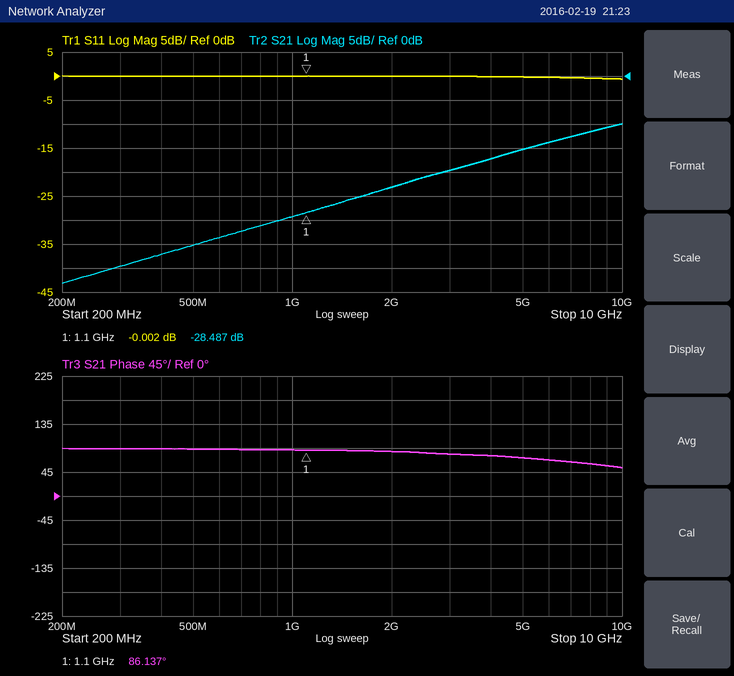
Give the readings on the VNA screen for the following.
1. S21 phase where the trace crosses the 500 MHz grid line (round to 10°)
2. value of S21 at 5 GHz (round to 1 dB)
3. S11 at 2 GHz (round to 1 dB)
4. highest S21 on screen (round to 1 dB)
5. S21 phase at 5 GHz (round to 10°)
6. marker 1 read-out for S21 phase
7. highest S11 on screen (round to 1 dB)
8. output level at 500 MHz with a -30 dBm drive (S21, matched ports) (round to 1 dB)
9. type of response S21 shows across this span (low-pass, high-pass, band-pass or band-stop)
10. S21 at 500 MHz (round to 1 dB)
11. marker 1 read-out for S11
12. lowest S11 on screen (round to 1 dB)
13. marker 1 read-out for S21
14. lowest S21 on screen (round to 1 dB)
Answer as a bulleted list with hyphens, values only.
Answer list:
- 90°
- -15 dB
- 0 dB
- -10 dB
- 70°
- 86.137°
- 0 dB
- -65 dBm
- high-pass
- -35 dB
- -0.002 dB
- -1 dB
- -28.487 dB
- -43 dB
